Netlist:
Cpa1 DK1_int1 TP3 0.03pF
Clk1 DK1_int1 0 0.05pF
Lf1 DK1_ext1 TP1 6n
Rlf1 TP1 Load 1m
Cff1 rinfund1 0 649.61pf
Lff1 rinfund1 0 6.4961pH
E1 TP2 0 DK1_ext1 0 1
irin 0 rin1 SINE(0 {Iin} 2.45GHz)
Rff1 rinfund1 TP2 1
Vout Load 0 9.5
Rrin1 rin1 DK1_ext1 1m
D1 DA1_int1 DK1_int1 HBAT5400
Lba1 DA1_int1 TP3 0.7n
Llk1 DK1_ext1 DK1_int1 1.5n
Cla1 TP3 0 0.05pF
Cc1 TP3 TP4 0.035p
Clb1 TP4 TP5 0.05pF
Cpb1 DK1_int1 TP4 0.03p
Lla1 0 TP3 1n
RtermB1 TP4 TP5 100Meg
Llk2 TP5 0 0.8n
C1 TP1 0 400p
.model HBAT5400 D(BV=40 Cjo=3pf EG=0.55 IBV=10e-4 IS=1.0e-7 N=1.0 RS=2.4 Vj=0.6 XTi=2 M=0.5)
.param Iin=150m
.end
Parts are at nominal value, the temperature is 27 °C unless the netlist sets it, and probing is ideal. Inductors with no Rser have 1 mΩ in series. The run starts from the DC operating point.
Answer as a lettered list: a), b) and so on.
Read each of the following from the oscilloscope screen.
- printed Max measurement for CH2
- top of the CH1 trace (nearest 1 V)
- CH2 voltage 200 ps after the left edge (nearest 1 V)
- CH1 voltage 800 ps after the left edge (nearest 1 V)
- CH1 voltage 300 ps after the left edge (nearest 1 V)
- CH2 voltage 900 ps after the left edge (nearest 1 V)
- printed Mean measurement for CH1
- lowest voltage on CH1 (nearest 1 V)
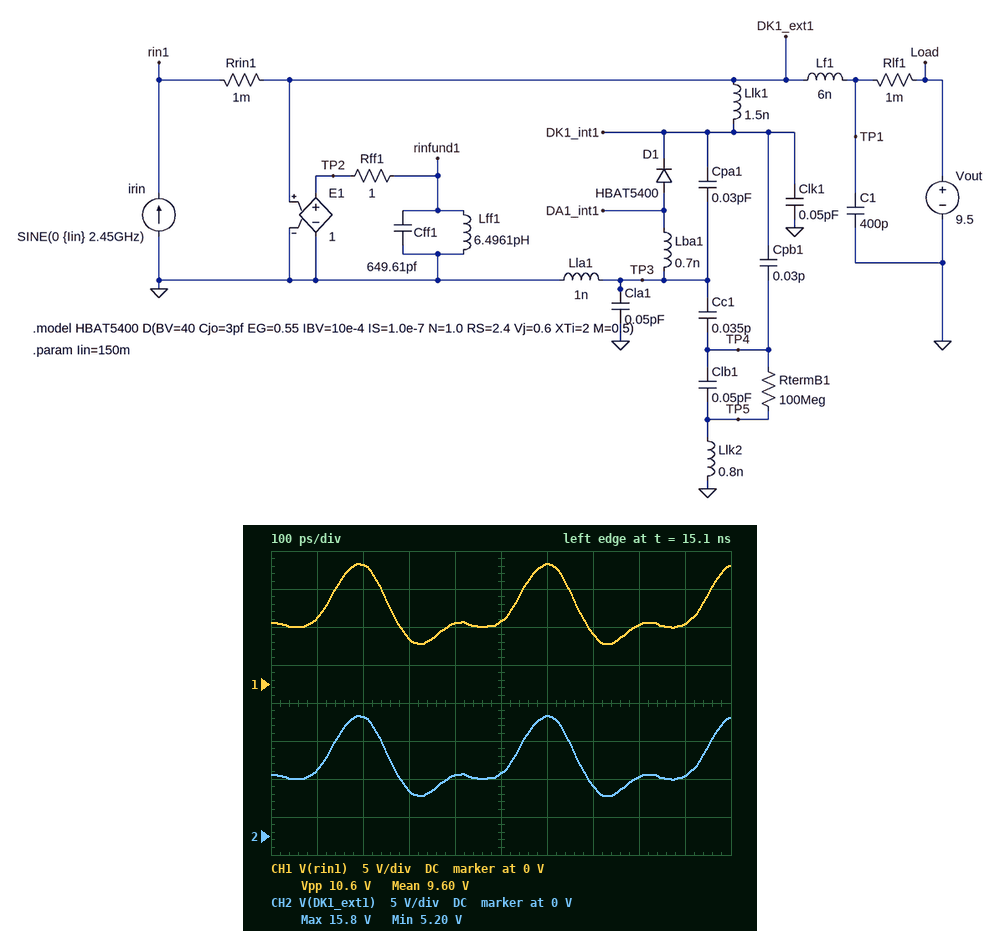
a) 15.8 V
b) 16 V
c) 16 V
d) 8 V
e) 6 V
f) 8 V
g) 9.60 V
h) 5 V
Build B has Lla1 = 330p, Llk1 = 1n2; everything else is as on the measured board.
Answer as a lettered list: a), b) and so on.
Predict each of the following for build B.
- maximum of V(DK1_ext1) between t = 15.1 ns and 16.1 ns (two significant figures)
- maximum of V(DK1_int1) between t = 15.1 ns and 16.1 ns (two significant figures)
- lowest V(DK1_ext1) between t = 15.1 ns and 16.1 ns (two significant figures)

a) 20 V
b) 24 V
c) 2.8 V
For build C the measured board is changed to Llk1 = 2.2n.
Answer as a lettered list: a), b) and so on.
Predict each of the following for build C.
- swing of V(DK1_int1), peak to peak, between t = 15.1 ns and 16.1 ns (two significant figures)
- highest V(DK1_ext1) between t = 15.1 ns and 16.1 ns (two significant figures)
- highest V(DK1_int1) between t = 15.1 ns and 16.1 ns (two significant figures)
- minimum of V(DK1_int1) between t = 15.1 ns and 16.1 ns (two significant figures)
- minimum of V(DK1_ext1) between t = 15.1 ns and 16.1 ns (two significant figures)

a) 16 V
b) 13 V
c) 20 V
d) 3.5 V
e) 7.1 V
